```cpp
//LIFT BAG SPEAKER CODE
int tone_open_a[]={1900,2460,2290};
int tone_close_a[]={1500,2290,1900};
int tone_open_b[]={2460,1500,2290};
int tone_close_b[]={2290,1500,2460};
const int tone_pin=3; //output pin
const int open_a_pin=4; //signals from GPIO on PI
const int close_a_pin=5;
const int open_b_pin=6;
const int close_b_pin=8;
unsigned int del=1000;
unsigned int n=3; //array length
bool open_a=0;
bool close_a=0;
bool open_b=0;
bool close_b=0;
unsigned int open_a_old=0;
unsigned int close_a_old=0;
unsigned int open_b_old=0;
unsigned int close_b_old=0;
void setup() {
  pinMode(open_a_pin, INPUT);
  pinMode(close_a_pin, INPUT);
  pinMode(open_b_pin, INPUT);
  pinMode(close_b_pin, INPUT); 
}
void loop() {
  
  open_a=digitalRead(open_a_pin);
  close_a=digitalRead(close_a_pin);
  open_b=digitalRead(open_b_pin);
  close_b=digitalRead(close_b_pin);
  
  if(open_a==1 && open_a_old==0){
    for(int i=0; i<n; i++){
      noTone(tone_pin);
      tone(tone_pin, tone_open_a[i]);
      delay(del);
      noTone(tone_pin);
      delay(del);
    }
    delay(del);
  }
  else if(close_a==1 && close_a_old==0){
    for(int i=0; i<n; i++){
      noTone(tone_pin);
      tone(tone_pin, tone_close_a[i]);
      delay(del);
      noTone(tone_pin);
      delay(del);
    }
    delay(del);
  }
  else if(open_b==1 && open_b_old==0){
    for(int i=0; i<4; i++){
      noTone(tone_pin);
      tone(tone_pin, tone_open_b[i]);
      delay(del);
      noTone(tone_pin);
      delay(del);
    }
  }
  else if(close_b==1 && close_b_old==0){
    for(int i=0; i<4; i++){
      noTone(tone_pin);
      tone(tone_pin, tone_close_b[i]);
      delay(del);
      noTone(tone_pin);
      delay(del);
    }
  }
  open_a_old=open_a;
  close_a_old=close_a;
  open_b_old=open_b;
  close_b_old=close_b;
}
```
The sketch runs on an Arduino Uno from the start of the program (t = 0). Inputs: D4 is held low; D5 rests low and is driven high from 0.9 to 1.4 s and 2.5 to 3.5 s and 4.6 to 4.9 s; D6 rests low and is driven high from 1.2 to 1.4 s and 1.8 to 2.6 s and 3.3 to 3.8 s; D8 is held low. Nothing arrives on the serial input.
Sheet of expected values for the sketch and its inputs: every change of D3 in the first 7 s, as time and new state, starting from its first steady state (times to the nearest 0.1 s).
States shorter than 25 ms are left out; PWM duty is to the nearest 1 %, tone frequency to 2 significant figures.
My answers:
0.9 s tone 1500 Hz; 1.9 s low; 2.9 s tone 2300 Hz; 3.9 s low; 4.9 s tone 1900 Hz; 5.9 s low
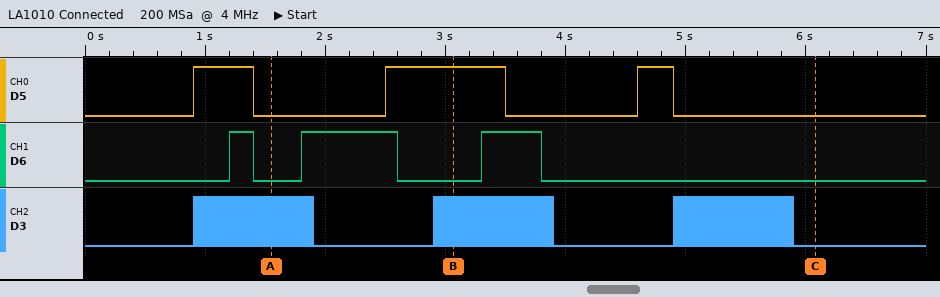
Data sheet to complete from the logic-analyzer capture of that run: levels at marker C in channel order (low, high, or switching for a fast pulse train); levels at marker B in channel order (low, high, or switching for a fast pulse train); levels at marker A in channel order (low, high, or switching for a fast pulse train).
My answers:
D5 low, D6 low, D3 low
D5 high, D6 low, D3 switching
D5 low, D6 low, D3 switching
